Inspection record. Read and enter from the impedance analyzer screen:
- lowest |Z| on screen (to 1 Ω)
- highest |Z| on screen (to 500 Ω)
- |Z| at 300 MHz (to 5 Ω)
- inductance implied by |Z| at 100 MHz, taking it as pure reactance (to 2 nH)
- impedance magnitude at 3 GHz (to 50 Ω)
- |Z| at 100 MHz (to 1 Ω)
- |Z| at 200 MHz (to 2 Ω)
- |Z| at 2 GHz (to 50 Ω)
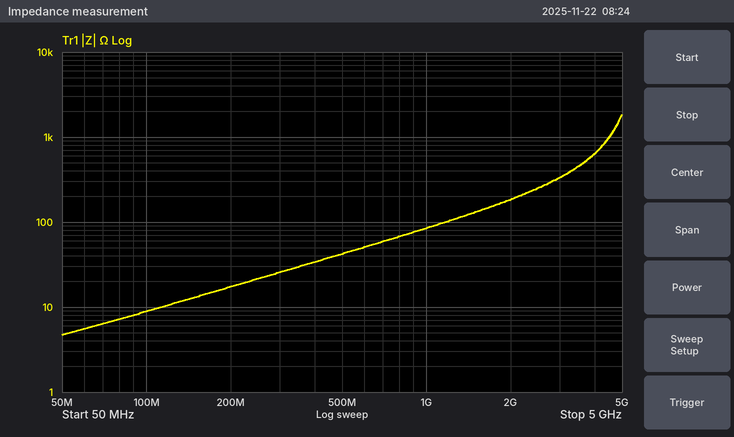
5 Ω
2.0 kΩ
25 Ω
14 nH
350 Ω
9 Ω
18 Ω
200 Ω
